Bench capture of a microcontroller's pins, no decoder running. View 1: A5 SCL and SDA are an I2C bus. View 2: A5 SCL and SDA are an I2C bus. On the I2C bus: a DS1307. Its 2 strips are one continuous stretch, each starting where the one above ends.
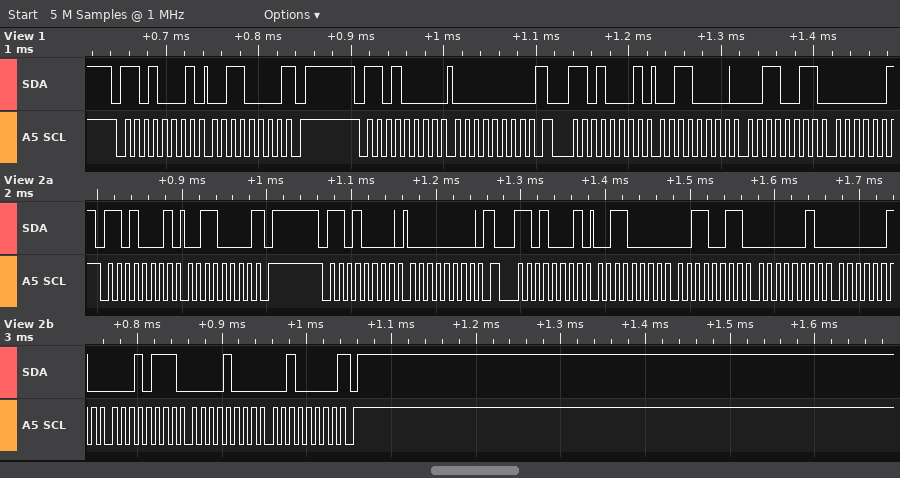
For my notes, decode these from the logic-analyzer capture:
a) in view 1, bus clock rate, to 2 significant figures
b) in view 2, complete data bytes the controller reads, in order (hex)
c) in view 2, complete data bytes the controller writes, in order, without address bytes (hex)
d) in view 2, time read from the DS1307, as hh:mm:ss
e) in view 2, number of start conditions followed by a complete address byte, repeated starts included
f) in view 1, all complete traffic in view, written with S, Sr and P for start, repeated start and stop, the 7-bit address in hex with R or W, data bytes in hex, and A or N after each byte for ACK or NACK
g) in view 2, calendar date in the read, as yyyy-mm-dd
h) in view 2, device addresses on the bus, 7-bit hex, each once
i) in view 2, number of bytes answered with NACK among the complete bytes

100 kHz
30 30 33 02 02 17 08 20
00
02:33:30
3
S 68R A 30 N P S 68W A 00 A Sr 68R A 30 A 33 A
2020-08-17
0x68
2
